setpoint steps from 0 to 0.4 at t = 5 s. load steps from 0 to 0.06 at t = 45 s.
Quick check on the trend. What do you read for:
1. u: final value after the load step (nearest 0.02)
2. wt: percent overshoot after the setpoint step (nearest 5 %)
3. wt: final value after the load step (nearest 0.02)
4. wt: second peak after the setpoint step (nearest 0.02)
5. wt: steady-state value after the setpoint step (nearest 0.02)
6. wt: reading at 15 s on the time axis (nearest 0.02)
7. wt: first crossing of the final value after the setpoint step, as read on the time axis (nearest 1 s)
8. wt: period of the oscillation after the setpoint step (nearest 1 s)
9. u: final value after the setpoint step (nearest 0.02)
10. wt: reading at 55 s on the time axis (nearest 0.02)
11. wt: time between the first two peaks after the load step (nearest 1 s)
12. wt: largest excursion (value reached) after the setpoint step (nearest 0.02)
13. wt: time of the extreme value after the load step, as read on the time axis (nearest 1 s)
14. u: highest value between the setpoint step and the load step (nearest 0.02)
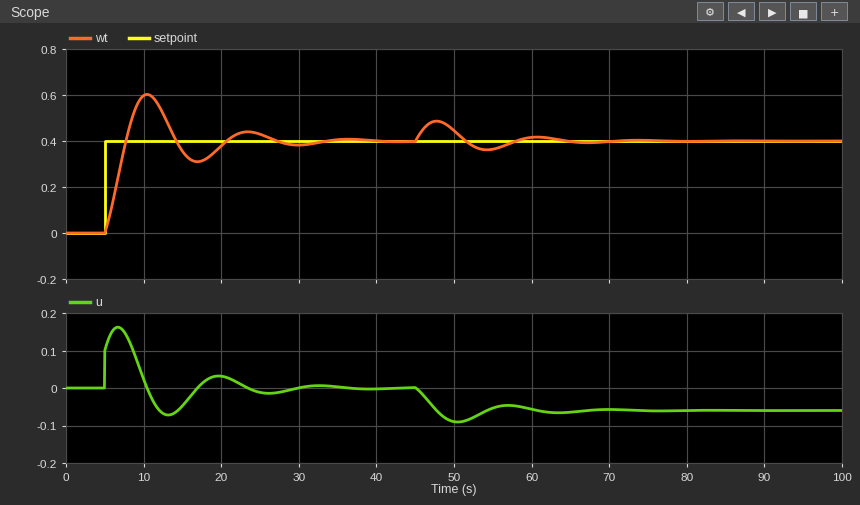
-0.06
50 %
0.40
0.44
0.40
0.36
8 s
13 s
0.00
0.36
13 s
0.60
48 s
0.16
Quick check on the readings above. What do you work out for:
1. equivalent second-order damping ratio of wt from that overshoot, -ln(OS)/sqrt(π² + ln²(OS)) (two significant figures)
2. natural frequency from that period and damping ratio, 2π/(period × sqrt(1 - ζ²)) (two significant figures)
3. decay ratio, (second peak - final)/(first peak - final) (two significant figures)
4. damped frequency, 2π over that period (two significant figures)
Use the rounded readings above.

0.22
0.50 rad/s
0.20
0.48 rad/s
